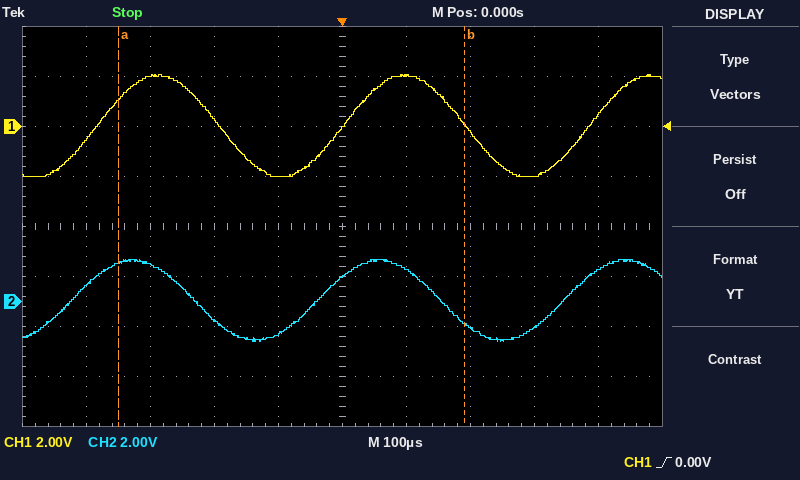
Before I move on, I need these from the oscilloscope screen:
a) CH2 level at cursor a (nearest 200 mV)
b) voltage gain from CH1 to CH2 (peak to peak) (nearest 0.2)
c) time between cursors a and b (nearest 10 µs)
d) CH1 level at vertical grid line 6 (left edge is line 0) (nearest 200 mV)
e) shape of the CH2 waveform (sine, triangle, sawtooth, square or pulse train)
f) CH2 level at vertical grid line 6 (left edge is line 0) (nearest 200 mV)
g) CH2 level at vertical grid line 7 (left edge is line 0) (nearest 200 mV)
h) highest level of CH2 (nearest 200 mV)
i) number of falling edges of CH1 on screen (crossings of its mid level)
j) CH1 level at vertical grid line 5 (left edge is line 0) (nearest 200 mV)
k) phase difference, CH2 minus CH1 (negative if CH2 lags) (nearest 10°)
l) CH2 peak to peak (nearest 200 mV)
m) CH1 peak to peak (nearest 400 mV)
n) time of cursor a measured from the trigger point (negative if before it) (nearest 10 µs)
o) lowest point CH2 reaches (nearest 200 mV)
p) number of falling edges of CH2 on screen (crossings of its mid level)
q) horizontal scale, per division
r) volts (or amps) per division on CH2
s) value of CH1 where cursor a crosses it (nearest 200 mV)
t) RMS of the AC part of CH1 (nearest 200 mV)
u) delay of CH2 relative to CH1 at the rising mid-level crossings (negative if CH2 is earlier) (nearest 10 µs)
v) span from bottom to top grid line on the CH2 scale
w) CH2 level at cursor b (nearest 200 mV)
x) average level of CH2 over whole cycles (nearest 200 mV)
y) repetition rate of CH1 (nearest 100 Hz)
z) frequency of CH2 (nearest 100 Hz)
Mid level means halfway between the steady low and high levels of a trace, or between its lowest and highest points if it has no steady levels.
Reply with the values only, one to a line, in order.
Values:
1.6 V
0.8
540 µs
2.0 V
sine
1.2 V
-1.0 V
1.6 V
2
0.0 V
+40°
3.2 V
4.0 V
-350 µs
-1.6 V
2
100 µs
2 V
1.0 V
1.4 V
-40 µs
16 V
-800 mV
0.0 V
2.6 kHz
2.6 kHz
